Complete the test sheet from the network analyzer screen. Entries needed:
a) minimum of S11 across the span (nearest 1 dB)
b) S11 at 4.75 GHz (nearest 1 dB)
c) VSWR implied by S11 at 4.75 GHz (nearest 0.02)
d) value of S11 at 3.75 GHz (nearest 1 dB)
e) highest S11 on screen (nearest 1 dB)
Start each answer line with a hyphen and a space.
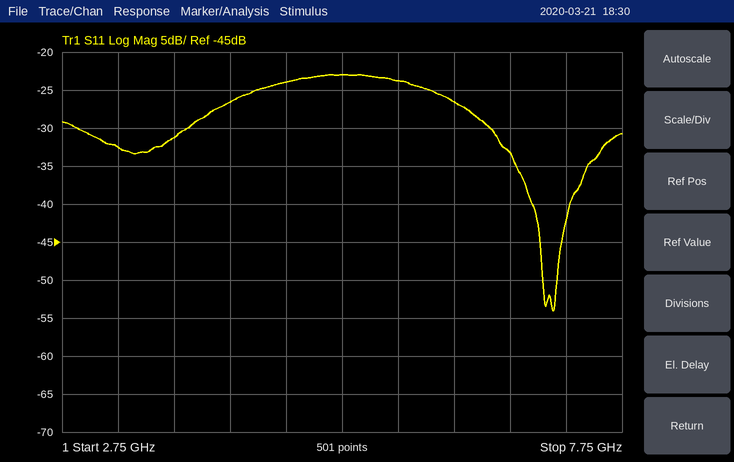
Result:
- -54 dB
- -24 dB
- 1.14
- -31 dB
- -23 dB
